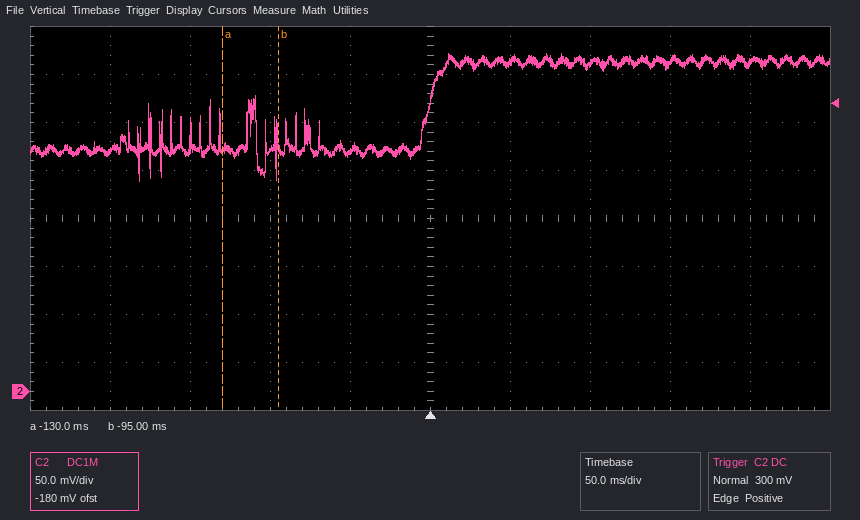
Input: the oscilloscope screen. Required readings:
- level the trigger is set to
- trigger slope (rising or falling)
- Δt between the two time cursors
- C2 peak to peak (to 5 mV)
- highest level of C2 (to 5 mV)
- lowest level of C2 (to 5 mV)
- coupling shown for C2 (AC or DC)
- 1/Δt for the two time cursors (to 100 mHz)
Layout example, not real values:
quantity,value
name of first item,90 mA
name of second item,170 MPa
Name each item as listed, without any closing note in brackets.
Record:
quantity,value
level the trigger is set to,300 mV
trigger slope,rising
Δt between the two time cursors,35 ms
C2 peak to peak,130 mV
highest level of C2,350 mV
lowest level of C2,220 mV
coupling shown for C2,DC
1/Δt for the two time cursors,28.6 Hz
